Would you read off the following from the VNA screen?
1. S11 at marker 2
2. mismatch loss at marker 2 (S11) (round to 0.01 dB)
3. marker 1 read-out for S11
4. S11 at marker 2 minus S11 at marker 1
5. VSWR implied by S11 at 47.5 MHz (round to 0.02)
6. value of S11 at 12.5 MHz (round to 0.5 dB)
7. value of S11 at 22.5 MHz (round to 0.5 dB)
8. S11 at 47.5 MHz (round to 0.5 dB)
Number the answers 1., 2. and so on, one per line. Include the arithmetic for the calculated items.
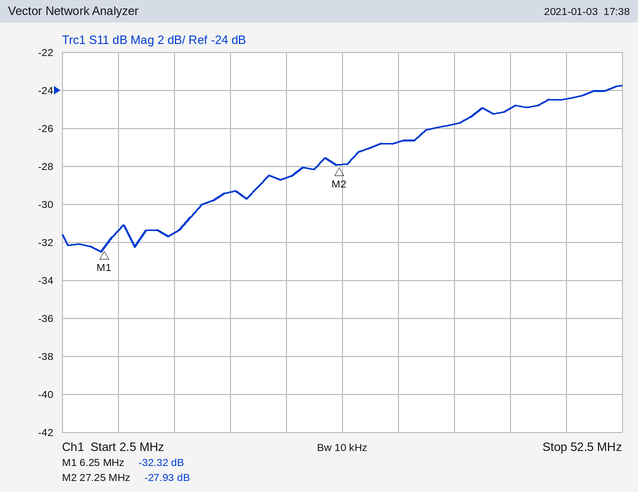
1. -27.93 dB
2. −10 log10(1 − 10^(-27.93/10)) ≈ 0.01 dB
3. -32.32 dB
4. -27.93 − (-32.32) = 4.39 dB
5. |Γ| = 10^(-24.5/20) = 0.0596; VSWR = (1 + 0.0596)/(1 − 0.0596) ≈ 1.13, so 1.12 to the nearest 0.02
6. -31.5 dB
7. -28.5 dB
8. -24.5 dB
